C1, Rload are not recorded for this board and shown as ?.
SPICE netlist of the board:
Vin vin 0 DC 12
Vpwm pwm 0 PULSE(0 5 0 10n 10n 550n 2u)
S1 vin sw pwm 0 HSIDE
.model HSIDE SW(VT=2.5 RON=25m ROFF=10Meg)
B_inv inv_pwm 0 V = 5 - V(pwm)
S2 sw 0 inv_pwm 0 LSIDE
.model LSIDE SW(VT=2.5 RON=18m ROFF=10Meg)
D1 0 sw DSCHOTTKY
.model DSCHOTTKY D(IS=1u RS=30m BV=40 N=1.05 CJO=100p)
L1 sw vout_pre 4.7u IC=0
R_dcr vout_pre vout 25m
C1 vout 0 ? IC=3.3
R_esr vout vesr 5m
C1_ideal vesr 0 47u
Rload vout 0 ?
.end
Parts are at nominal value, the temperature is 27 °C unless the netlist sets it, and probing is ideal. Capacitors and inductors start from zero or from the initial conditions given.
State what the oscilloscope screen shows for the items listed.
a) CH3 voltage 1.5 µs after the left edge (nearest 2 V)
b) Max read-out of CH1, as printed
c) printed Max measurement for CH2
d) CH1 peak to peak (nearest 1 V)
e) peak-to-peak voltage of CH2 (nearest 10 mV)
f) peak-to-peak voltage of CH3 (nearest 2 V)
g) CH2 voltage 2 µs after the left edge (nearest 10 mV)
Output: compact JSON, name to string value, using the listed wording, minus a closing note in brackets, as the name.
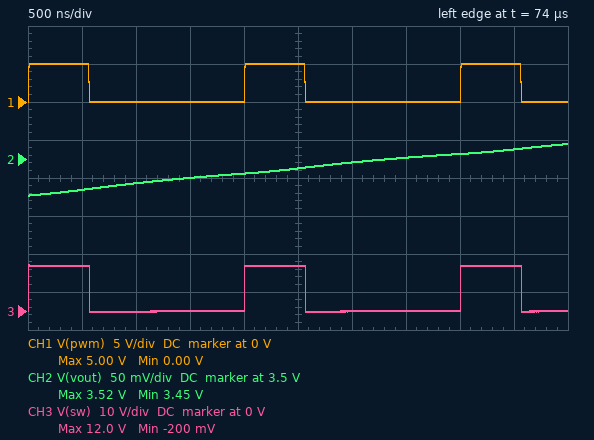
{"CH3 voltage 1.5 µs after the left edge": "0 V", "Max read-out of CH1, as printed": "5.00 V", "printed Max measurement for CH2": "3.52 V", "CH1 peak to peak": "5 V", "peak-to-peak voltage of CH2": "70 mV", "peak-to-peak voltage of CH3": "12 V", "CH2 voltage 2 µs after the left edge": "3.48 V"}
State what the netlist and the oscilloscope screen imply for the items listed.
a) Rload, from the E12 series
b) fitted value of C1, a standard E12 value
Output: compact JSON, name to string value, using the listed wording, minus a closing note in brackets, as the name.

{"Rload, from the E12 series": "0.68 Ω", "fitted value of C1, a standard E12 value": "100 µF"}
